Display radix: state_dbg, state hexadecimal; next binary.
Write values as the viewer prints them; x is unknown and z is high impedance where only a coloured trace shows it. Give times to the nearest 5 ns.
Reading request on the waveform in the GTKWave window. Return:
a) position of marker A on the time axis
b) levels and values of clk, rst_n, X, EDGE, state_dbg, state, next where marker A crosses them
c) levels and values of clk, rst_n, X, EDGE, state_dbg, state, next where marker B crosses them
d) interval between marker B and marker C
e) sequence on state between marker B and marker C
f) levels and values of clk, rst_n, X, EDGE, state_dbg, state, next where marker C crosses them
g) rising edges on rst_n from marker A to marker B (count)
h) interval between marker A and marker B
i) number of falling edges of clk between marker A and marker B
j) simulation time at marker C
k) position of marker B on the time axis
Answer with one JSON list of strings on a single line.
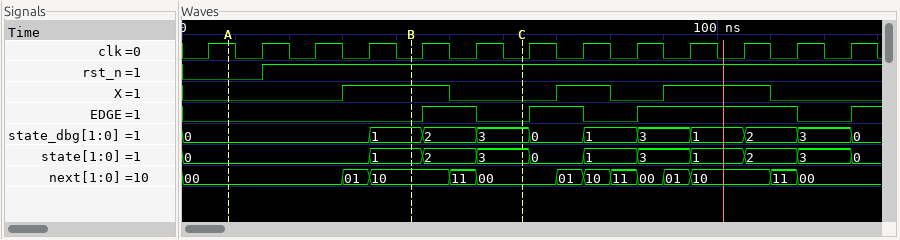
["10 ns", "clk=1, rst_n=0, X=0, EDGE=0, state_dbg=0, state=0, next=00", "clk=0, rst_n=1, X=1, EDGE=0, state_dbg=1, state=1, next=10", "20 ns", "1, 2, 3", "clk=0, rst_n=1, X=0, EDGE=0, state_dbg=3, state=3, next=00", "1", "35 ns", "4", "65 ns", "45 ns"]
